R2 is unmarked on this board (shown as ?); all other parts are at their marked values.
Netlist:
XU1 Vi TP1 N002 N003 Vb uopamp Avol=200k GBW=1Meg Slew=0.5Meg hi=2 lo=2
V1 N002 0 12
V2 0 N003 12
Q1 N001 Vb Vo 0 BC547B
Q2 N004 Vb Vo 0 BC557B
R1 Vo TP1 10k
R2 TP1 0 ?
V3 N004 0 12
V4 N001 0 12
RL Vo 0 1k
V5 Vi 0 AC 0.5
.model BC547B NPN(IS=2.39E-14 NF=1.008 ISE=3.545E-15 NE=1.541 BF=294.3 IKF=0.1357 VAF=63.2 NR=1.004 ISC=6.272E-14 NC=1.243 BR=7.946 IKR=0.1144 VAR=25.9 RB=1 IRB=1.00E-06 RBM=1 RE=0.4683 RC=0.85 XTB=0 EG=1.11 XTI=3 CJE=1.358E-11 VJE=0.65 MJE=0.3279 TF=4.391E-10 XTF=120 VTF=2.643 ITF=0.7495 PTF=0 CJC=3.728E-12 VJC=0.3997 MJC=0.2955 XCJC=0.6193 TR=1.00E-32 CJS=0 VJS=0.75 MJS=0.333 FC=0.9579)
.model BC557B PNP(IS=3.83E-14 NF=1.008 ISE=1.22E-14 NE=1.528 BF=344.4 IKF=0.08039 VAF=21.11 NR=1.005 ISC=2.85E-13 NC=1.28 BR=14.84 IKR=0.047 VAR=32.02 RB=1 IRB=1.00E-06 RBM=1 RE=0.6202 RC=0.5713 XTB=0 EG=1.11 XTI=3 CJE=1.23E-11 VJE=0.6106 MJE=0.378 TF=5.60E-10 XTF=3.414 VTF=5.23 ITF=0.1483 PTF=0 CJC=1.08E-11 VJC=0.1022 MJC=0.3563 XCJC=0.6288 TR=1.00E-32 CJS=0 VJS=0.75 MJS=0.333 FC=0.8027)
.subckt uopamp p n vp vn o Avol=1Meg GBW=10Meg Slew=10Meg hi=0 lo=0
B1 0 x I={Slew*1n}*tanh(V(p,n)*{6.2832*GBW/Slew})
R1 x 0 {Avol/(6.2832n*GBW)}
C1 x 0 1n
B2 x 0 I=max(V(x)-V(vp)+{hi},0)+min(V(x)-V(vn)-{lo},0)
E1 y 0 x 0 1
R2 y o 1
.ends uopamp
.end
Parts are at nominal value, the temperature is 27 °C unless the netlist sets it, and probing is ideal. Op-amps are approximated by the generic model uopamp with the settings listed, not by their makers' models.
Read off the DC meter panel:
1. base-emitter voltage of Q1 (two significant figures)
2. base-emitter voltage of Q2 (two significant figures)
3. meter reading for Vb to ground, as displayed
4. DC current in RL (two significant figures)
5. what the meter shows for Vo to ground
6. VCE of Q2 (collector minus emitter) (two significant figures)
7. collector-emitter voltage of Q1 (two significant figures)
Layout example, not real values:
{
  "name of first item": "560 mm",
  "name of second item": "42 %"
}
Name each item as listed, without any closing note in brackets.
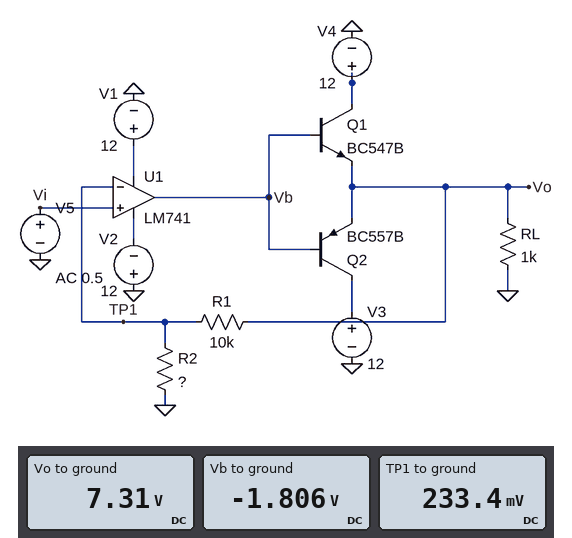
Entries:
{
  "base-emitter voltage of Q1": "-9.1 V",
  "base-emitter voltage of Q2": "-9.1 V",
  "meter reading for Vb to ground, as displayed": "-1.806 V",
  "DC current in RL": "7.3 mA",
  "what the meter shows for Vo to ground": "7.31 V",
  "VCE of Q2 (collector minus emitter)": "4.7 V",
  "collector-emitter voltage of Q1": "4.7 V"
}
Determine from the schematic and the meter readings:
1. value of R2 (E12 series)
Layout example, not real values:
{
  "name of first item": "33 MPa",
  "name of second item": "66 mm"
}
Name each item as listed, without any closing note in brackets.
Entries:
{
  "value of R2": "330 Ω"
}
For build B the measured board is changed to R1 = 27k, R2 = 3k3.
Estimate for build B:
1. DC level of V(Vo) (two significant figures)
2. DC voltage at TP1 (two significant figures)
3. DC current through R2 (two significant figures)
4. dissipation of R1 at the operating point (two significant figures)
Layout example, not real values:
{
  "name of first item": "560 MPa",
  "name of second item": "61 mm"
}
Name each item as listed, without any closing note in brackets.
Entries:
{
  "DC level of V(Vo)": "7.3 V",
  "DC voltage at TP1": "800 mV",
  "DC current through R2": "240 µA",
  "dissipation of R1 at the operating point": "1.6 mW"
}
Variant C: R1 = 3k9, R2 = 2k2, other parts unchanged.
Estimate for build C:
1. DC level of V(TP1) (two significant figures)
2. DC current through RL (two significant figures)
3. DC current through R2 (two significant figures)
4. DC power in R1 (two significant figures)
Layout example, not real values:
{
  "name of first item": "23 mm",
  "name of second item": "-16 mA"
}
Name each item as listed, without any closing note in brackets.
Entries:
{
  "DC level of V(TP1)": "2.6 V",
  "DC current through RL": "7.3 mA",
  "DC current through R2": "1.2 mA",
  "DC power in R1": "5.6 mW"
}
